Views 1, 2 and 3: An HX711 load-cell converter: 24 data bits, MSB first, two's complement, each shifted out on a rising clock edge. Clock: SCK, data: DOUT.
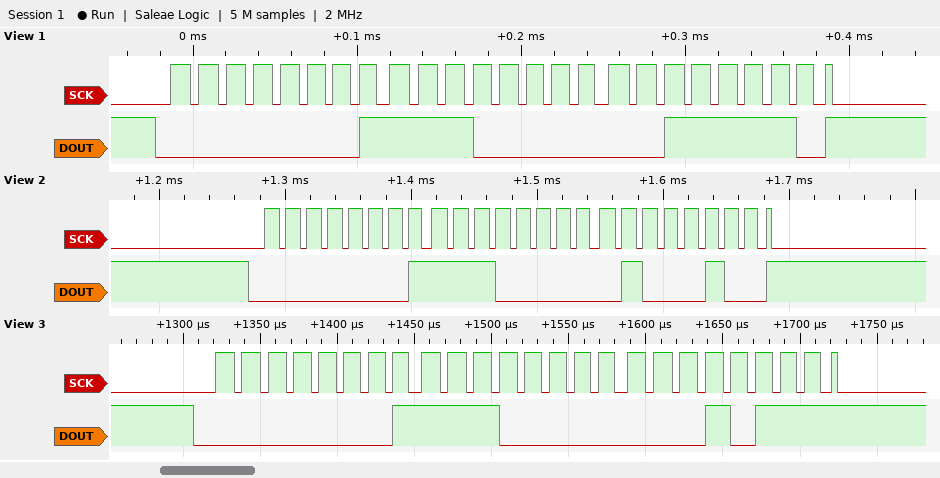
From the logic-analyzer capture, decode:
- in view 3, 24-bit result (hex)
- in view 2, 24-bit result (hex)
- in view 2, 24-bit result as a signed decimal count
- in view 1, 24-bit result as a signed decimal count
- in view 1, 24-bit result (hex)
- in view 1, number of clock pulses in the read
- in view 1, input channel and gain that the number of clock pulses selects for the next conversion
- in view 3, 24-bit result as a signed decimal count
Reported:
0x01E017
0x01E044
122948
122942
0x01E03E
25
channel A, gain 128
122903
